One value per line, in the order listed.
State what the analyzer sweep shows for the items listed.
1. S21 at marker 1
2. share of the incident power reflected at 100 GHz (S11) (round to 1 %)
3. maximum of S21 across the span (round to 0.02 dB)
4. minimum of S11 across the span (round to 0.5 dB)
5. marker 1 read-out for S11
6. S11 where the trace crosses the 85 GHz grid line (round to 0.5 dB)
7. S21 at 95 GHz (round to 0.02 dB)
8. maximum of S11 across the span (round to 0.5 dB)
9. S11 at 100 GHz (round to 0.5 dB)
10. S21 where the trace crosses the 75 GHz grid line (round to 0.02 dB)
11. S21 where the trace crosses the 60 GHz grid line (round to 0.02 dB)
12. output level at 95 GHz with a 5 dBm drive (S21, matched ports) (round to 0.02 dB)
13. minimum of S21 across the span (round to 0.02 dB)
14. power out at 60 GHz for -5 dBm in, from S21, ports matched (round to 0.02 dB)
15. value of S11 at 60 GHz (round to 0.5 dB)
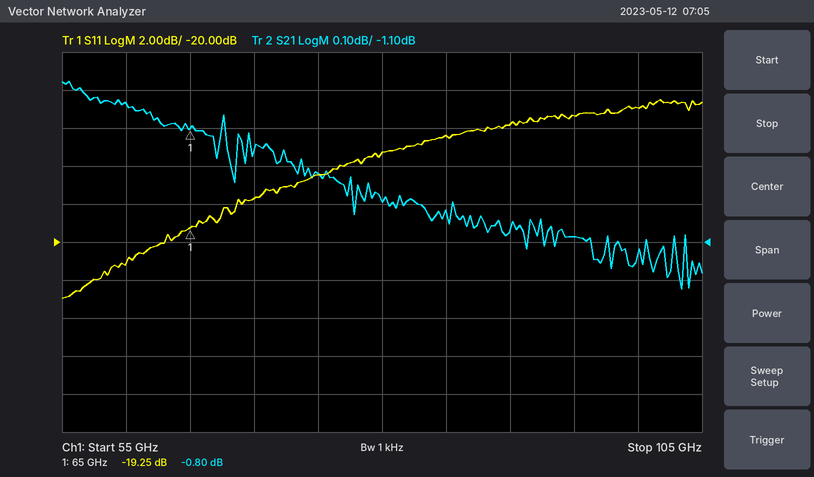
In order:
-0.80 dB
5 %
-0.68 dB
-23.0 dB
-19.25 dB
-14.5 dB
-1.08 dB
-12.5 dB
-13.0 dB
-0.92 dB
-0.74 dB
3.92 dBm
-1.22 dB
-5.74 dBm
-21.0 dB
